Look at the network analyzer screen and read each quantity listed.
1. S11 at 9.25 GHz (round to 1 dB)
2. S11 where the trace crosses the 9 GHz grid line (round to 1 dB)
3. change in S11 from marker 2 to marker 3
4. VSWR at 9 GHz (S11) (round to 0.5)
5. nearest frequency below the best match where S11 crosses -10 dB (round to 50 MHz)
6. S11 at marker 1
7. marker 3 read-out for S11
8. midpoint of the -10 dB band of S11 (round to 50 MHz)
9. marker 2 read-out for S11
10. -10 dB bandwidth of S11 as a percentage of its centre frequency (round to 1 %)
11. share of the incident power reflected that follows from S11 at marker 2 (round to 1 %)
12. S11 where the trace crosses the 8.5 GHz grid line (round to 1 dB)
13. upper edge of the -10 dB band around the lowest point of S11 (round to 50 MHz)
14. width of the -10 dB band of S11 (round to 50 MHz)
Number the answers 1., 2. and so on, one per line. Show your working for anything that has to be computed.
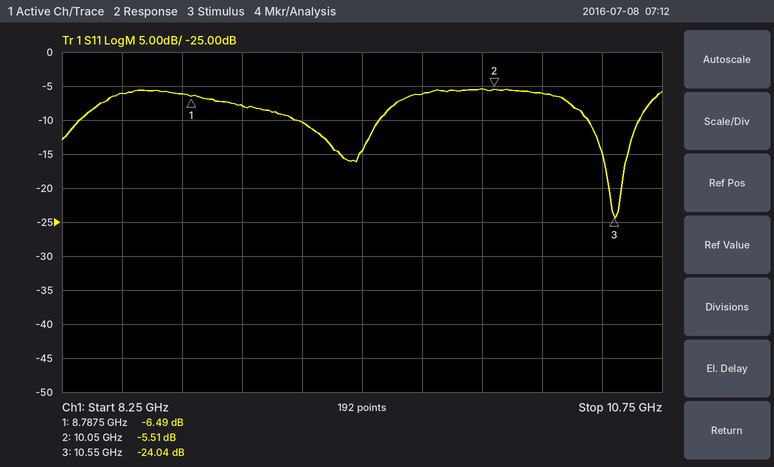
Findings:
1. -10 dB
2. -8 dB
3. -24.04 − (-5.51) = -18.53 dB
4. |Γ| = 10^(-8/20) = 0.3981; VSWR = (1 + 0.3981)/(1 − 0.3981) ≈ 2.32, so 2.5 to the nearest 0.5
5. 10.45 GHz
6. -6.49 dB
7. -24.04 dB
8. 10.55 GHz
9. -5.51 dB
10. 200 MHz / 10.55 GHz ≈ 2 %
11. 10^(-5.51/10) ≈ 28 %
12. -6 dB
13. 10.65 GHz
14. 10.65 GHz − 10.45 GHz = 200 MHz
